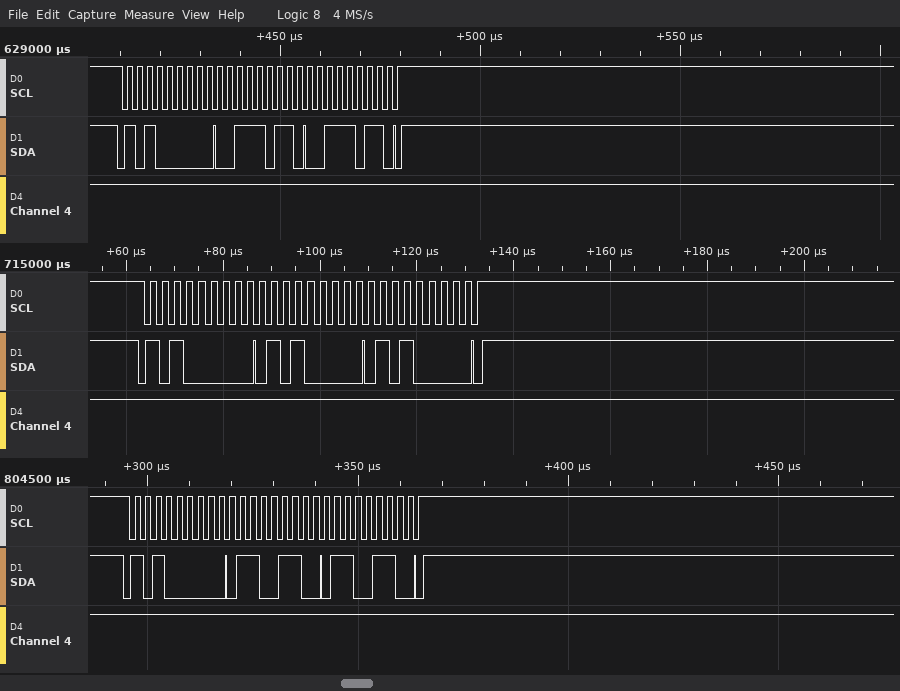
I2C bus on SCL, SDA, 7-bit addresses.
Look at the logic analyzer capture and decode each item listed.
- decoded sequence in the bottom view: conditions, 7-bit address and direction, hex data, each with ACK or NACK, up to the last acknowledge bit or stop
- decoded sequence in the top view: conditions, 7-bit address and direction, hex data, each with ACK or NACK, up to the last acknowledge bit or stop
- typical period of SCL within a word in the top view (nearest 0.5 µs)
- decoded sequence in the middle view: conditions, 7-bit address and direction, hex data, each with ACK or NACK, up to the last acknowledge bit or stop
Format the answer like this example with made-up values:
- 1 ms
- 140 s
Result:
- start, address 50 write ACK, 66 ACK, 66 ACK, stop
- start, address 50 write ACK, 3B ACK, 3B ACK, stop
- 2.5 µs
- start, address 50 write ACK, 50 ACK, 50 ACK, stop
